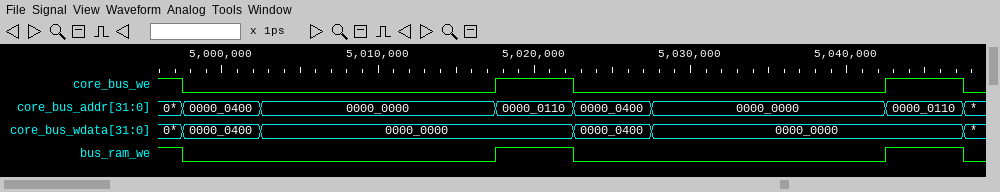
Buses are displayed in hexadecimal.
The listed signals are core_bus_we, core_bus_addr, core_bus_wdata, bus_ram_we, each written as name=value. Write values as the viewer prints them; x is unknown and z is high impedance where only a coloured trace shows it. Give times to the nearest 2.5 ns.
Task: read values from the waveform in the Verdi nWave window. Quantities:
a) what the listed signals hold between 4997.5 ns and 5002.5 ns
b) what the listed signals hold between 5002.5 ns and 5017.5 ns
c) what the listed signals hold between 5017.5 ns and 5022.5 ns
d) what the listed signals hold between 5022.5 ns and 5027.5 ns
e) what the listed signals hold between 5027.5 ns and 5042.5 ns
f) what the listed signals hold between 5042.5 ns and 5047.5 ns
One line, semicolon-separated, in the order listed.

core_bus_we=0, core_bus_addr=0000_0400, core_bus_wdata=0000_0400, bus_ram_we=0; core_bus_we=0, core_bus_addr=0000_0000, core_bus_wdata=0000_0000, bus_ram_we=0; core_bus_we=1, core_bus_addr=0000_0110, core_bus_wdata=0000_0000, bus_ram_we=1; core_bus_we=0, core_bus_addr=0000_0400, core_bus_wdata=0000_0400, bus_ram_we=0; core_bus_we=0, core_bus_addr=0000_0000, core_bus_wdata=0000_0000, bus_ram_we=0; core_bus_we=1, core_bus_addr=0000_0110, core_bus_wdata=0000_0000, bus_ram_we=1
